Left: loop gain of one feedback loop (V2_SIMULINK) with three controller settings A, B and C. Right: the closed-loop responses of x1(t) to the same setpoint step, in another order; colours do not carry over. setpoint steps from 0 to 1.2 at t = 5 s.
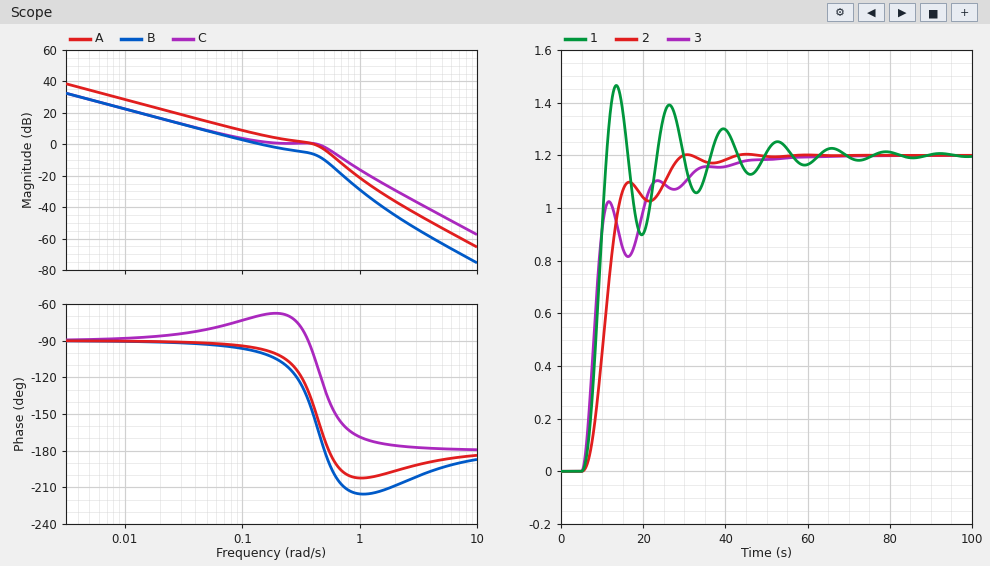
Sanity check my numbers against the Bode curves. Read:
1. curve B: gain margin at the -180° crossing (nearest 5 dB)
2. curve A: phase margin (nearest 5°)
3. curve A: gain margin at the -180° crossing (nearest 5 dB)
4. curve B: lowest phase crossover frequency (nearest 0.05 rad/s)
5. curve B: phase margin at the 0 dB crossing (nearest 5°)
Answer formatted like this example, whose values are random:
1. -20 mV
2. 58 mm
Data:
1. 10 dB
2. 35°
3. 5 dB
4. 0.50 rad/s
5. 80°
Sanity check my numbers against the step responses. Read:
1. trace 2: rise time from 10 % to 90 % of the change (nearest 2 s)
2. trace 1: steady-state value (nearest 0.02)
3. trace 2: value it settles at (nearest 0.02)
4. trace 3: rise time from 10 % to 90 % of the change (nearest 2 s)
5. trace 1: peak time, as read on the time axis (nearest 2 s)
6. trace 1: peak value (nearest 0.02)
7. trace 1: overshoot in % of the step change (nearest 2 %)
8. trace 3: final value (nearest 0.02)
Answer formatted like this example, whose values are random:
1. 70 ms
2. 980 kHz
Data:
1. 8 s
2. 1.20
3. 1.20
4. 16 s
5. 14 s
6. 1.46
7. 22 %
8. 1.20
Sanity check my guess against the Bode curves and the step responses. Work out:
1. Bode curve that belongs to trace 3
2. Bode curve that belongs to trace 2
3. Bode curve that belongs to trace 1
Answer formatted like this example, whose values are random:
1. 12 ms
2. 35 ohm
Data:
1. C
2. B
3. A
